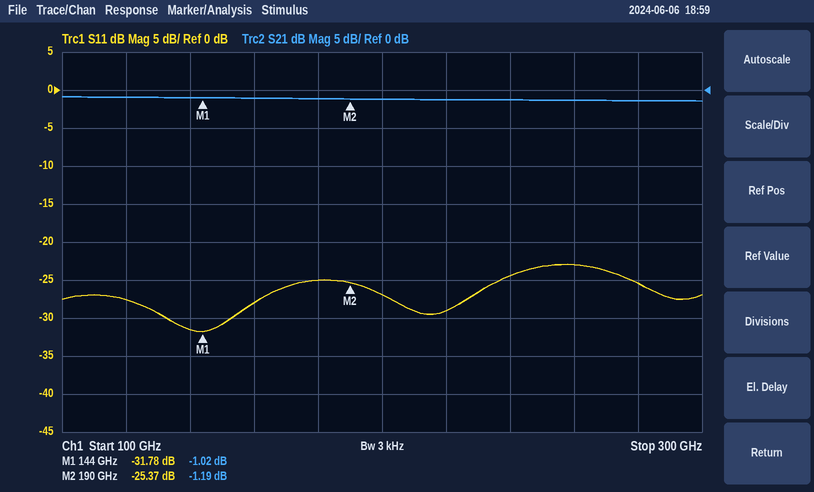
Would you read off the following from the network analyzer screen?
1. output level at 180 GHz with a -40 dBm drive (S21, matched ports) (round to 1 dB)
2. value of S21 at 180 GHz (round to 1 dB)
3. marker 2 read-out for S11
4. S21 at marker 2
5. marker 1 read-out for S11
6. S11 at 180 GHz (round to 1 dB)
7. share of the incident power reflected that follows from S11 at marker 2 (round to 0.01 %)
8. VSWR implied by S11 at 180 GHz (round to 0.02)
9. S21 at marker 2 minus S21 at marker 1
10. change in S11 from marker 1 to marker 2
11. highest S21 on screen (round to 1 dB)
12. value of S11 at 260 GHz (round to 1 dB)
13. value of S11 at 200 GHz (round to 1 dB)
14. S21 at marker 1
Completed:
-41 dBm
-1 dB
-25.37 dB
-1.19 dB
-31.78 dB
-25 dB
0.29 %
1.12
-0.17 dB
6.41 dB
-1 dB
-23 dB
-27 dB
-1.02 dB
